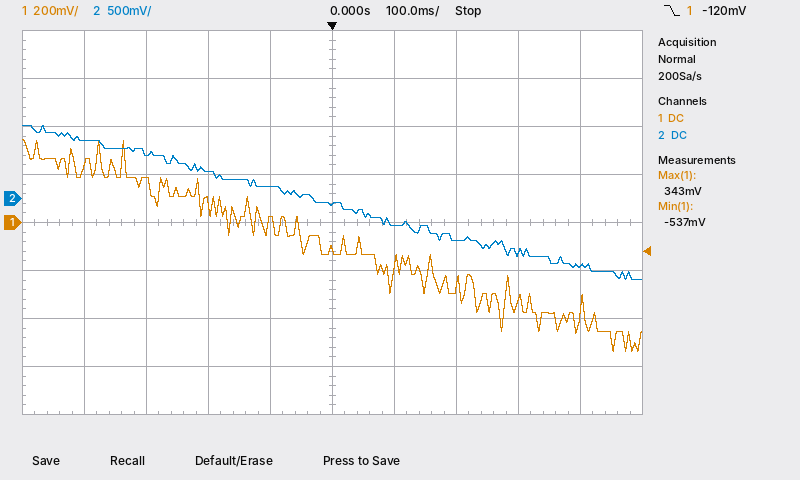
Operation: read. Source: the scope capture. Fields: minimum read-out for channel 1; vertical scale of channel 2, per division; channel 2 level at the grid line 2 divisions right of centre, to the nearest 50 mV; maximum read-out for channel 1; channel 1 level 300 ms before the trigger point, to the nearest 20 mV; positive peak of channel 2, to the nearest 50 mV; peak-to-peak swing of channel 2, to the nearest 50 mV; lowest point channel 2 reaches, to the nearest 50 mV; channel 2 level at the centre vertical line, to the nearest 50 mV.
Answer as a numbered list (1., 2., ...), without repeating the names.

1. -537 mV
2. 500 mV
3. -450 mV
4. 343 mV
5. 180 mV
6. 750 mV
7. 1.60 V
8. -850 mV
9. -50 mV
